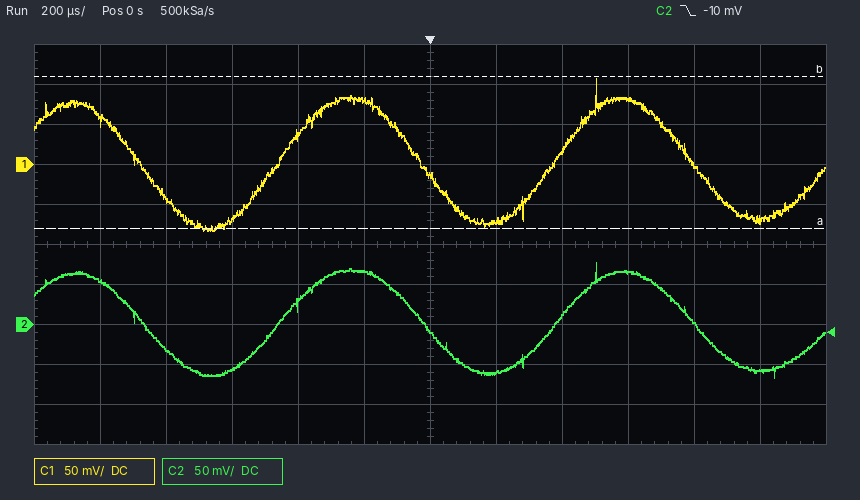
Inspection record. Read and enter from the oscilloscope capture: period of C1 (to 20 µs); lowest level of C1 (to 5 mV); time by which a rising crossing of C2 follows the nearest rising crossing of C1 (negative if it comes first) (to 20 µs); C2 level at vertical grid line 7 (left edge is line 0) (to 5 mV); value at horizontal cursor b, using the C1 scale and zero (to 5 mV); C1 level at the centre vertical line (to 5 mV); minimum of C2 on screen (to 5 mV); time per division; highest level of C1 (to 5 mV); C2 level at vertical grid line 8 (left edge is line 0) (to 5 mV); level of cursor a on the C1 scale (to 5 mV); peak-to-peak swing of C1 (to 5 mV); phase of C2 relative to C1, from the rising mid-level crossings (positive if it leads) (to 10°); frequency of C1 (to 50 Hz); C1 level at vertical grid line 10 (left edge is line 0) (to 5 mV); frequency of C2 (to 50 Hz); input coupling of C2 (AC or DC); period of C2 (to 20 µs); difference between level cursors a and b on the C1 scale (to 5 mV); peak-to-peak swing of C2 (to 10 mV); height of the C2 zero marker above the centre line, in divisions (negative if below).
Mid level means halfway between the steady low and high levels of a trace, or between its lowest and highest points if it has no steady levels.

840 µs
-80 mV
0 µs
-60 mV
110 mV
-15 mV
-65 mV
200 µs
110 mV
10 mV
-80 mV
190 mV
0°
1.20 kHz
0 mV
1.20 kHz
DC
840 µs
190 mV
140 mV
-2.0 div
